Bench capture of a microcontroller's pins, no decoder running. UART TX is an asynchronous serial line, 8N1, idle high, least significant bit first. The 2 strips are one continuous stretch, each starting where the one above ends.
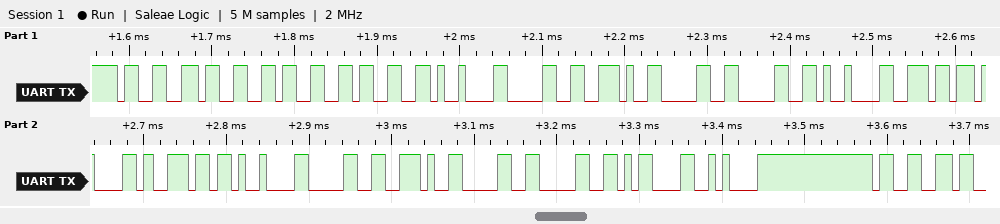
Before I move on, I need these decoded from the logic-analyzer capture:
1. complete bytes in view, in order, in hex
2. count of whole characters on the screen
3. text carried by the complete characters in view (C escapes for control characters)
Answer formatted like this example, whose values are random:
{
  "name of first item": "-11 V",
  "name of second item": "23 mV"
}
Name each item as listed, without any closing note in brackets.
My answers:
{
  "complete bytes in view, in order, in hex": "0x33 0x33 0x33 0x33 0x09 0x30 0x2E 0x30 0x30 0x09 0x6E 0x61 0x6E 0x09 0x30 0x2E 0x30 0x30 0x0D 0x0A 0x33",
  "count of whole characters on the screen": "21",
  "text carried by the complete characters in view": "\"3333\\t0.00\\tnan\\t0.00\\r\\n3\""
}
